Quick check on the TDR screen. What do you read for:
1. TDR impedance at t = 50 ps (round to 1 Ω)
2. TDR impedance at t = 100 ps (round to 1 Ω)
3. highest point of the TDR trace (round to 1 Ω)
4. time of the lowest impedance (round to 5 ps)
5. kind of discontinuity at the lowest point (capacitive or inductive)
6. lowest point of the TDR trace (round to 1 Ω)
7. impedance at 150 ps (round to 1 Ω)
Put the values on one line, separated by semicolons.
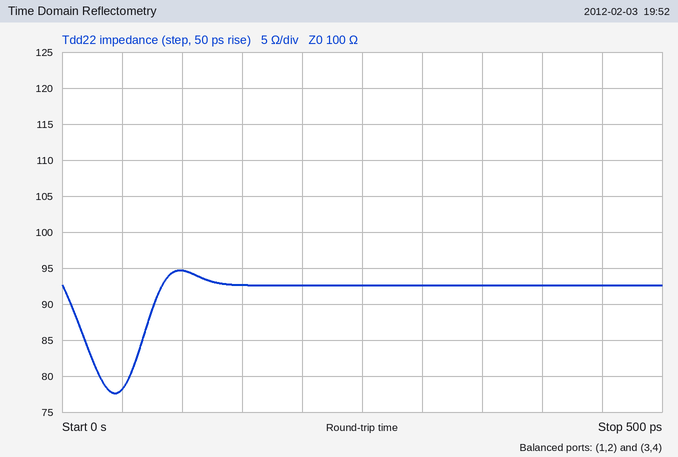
78 Ω; 95 Ω; 95 Ω; 45 ps; capacitive; 78 Ω; 93 Ω
